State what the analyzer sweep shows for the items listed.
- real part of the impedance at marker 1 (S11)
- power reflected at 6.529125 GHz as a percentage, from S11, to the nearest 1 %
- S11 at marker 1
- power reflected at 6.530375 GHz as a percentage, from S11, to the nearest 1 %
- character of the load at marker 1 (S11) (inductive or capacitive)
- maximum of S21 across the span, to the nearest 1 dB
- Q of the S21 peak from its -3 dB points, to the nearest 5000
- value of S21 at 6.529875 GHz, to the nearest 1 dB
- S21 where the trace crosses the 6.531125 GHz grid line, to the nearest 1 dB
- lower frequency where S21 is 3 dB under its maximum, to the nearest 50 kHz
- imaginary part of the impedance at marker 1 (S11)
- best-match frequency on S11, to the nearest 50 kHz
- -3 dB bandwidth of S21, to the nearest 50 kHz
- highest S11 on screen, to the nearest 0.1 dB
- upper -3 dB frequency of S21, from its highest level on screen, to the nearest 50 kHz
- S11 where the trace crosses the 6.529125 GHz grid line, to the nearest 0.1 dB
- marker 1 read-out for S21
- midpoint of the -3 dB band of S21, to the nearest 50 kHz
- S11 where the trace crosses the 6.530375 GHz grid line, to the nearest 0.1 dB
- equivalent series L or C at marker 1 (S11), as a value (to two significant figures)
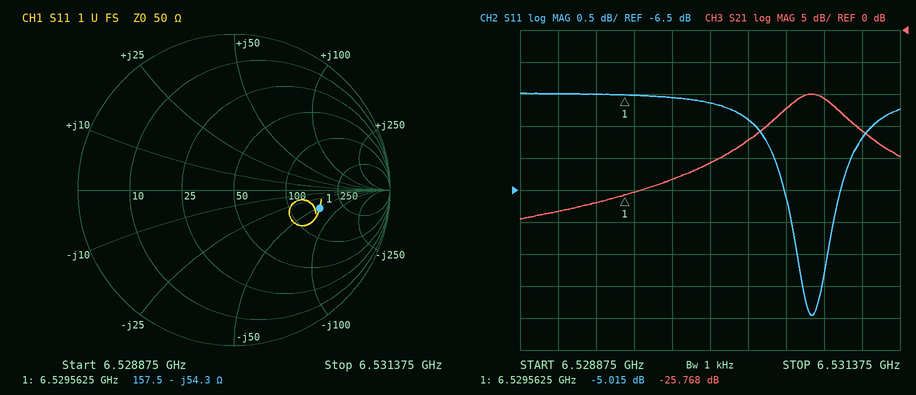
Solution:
157.5 Ω
32 %
-5.015 dB
29 %
capacitive
-10 dB
15000
-23 dB
-16 dB
6.53060 GHz
-54.3 Ω
6.53080 GHz
400 kHz
-5.0 dB
6.53100 GHz
-5.0 dB
-25.768 dB
6.53080 GHz
-5.4 dB
450 fF
